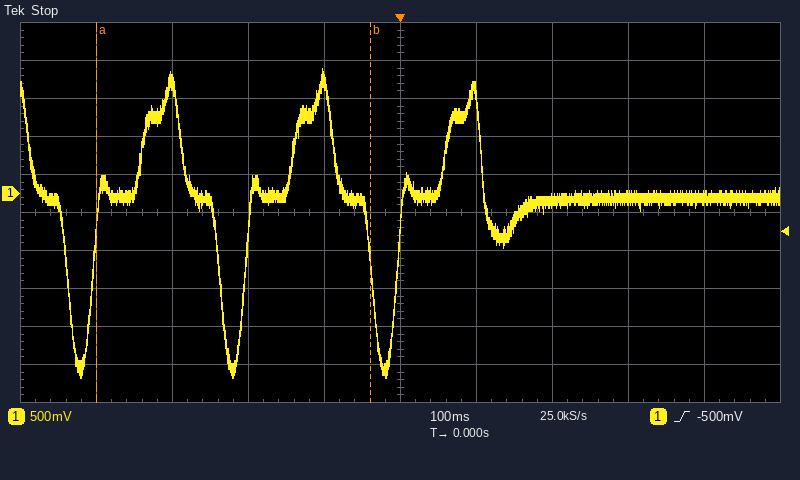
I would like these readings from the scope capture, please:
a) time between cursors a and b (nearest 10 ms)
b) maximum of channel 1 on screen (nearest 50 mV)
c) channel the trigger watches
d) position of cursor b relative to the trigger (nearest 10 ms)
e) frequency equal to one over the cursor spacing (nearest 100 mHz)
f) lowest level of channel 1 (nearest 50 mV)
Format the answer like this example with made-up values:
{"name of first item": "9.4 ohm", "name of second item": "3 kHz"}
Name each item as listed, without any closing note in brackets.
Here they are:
{"time between cursors a and b": "360 ms", "maximum of channel 1 on screen": "1.65 V", "channel the trigger watches": "channel 1", "position of cursor b relative to the trigger": "-40 ms", "frequency equal to one over the cursor spacing": "2.8 Hz", "lowest level of channel 1": "-2.45 V"}
